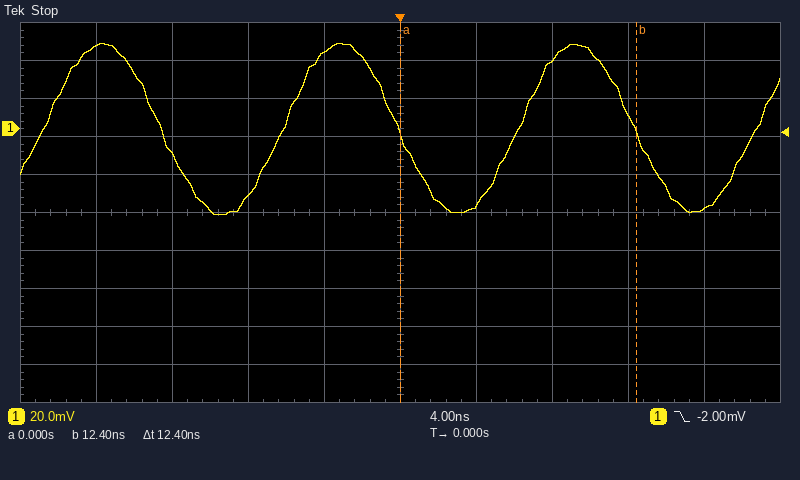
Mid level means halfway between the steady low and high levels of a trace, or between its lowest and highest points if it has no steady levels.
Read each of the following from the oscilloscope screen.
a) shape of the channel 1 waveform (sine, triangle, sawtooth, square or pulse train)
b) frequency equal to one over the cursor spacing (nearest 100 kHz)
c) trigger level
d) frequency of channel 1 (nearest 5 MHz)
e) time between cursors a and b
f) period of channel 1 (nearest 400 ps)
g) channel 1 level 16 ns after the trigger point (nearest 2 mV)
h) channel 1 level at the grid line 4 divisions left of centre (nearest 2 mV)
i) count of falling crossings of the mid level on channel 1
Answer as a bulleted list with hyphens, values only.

- sine
- 80.6 MHz
- -2.00 mV
- 80 MHz
- 12.4 ns
- 12.4 ns
- -42 mV
- 44 mV
- 3
